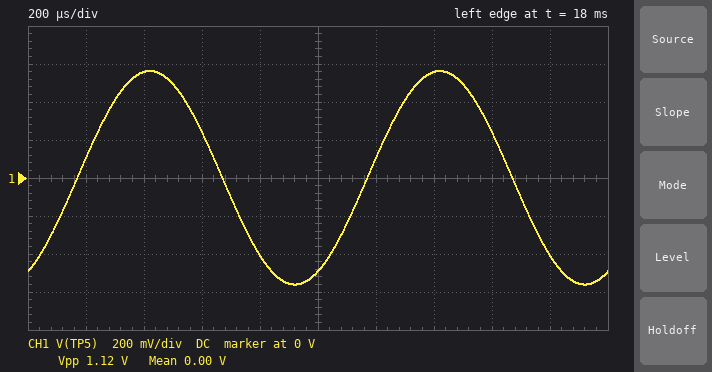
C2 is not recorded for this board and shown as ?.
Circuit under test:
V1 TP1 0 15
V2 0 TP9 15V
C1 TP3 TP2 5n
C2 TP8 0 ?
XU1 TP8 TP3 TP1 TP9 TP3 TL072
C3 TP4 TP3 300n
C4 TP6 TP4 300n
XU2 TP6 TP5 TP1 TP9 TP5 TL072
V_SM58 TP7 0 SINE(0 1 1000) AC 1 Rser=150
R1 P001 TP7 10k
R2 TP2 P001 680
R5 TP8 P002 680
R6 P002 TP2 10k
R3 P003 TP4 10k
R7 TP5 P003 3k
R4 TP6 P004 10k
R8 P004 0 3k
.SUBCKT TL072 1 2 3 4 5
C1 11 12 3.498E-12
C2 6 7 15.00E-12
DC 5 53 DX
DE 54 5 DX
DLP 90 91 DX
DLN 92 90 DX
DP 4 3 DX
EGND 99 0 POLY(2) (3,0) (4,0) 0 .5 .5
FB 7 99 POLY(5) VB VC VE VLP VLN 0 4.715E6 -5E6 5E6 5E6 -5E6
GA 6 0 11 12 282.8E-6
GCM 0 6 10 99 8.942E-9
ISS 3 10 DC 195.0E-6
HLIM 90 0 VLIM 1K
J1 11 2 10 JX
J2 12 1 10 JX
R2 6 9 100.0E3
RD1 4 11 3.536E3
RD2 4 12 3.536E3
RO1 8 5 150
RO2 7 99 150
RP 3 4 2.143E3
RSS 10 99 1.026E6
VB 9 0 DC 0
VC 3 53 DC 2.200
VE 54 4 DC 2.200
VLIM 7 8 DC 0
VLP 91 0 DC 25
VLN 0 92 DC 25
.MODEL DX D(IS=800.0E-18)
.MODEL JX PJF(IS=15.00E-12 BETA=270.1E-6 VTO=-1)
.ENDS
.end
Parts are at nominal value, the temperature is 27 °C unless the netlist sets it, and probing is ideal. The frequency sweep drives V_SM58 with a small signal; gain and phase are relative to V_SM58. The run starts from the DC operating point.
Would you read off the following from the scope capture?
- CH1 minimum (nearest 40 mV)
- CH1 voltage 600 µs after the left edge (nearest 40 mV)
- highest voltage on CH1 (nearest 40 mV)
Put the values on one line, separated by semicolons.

-560 mV; 240 mV; 560 mV
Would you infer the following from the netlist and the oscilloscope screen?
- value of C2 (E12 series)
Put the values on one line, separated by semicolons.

12 nF
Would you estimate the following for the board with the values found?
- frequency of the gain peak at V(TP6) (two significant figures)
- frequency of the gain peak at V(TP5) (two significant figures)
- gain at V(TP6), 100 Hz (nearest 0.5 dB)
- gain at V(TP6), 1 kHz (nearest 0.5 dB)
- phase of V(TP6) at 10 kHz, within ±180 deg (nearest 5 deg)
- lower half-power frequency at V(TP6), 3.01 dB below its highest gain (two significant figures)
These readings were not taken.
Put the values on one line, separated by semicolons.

200 Hz; 200 Hz; -1.5 dB; -5.0 dB; -150 deg; 56 Hz
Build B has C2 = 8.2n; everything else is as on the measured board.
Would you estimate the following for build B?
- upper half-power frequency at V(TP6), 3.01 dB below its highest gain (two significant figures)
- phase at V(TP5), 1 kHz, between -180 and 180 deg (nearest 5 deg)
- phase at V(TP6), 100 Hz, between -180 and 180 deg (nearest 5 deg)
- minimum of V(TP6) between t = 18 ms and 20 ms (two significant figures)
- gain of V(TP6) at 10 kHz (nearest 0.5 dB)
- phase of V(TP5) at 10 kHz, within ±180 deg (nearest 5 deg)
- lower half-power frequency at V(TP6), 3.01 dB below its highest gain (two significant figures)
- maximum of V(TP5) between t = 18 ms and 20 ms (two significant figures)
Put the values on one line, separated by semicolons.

1.2 kHz; -50 deg; 40 deg; -730 mV; -26.5 dB; -150 deg; 58 Hz; 730 mV
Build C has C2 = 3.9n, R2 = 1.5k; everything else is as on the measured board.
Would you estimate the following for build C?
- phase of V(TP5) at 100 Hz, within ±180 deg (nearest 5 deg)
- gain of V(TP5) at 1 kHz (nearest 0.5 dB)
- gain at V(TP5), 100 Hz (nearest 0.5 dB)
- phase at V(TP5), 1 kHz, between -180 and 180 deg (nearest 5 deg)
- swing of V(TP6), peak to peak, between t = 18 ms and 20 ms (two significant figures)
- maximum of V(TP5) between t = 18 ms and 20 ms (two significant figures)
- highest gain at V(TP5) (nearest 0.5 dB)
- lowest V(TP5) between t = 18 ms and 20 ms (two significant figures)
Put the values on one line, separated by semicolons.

40 deg; -0.5 dB; -1.5 dB; -25 deg; 1.9 V; 950 mV; 0 dB; -940 mV
